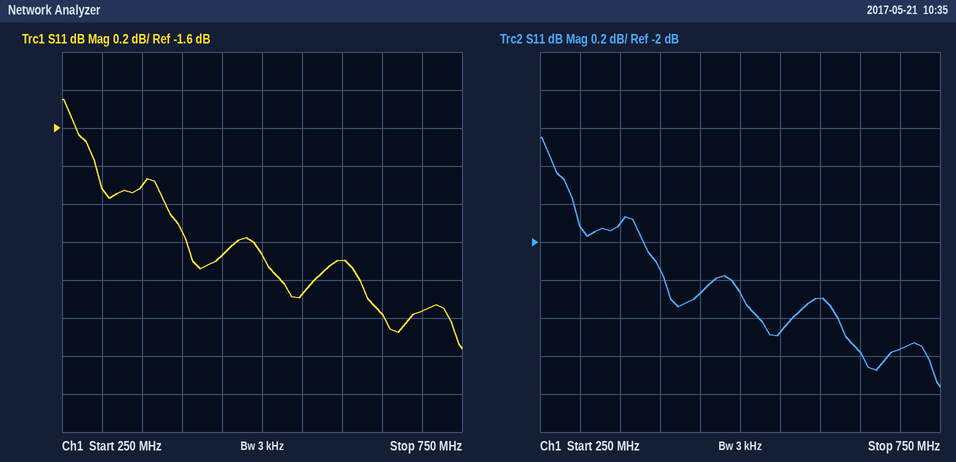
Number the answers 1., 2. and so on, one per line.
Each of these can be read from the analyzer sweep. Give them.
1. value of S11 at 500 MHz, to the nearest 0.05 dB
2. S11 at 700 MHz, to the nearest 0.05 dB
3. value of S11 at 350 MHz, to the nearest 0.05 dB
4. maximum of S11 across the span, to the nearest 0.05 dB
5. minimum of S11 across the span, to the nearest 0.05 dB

1. -2.25 dB
2. -2.55 dB
3. -1.90 dB
4. -1.45 dB
5. -2.75 dB
